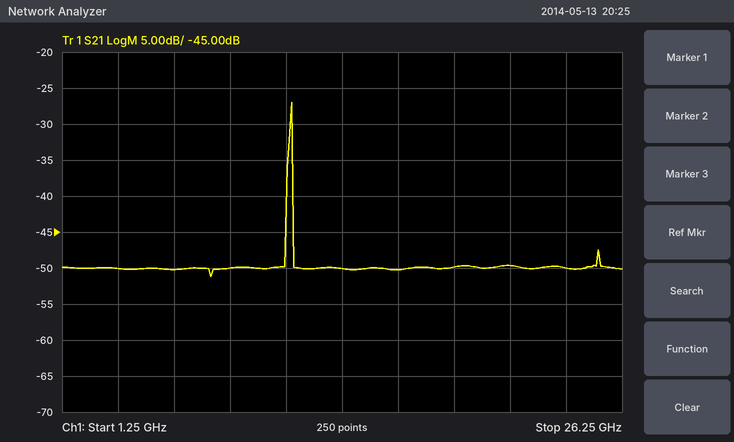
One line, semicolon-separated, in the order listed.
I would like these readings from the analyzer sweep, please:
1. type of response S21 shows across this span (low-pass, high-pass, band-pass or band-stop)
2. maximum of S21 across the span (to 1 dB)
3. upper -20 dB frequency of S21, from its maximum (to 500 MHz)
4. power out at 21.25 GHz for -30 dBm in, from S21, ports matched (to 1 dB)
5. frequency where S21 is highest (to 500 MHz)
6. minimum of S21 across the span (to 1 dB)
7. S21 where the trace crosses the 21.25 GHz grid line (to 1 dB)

band-pass; -27 dB; 11.5 GHz; -80 dBm; 11.5 GHz; -51 dB; -50 dB
